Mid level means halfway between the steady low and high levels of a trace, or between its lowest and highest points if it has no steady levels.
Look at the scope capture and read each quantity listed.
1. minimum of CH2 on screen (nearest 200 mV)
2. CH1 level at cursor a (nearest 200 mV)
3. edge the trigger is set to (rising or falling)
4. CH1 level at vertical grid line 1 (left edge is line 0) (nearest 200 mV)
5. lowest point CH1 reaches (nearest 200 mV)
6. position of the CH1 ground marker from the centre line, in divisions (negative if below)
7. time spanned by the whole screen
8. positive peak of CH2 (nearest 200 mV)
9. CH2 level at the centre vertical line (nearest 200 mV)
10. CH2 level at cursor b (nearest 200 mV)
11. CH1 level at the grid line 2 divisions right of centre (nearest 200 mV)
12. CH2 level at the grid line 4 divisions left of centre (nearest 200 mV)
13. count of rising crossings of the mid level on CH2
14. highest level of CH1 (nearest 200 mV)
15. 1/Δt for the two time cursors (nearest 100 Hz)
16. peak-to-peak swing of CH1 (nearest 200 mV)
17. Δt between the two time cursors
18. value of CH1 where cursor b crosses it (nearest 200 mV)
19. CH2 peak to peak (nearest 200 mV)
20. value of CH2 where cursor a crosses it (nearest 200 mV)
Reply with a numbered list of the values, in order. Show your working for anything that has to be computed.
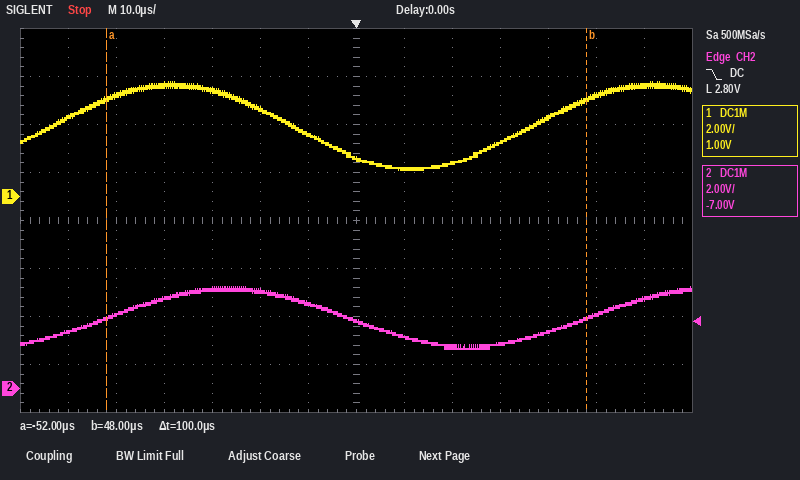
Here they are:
1. 1.6 V
2. 4.0 V
3. falling
4. 3.2 V
5. 1.2 V
6. +0.5 div
7. 140 µs
8. 4.2 V
9. 2.8 V
10. 3.0 V
11. 1.4 V
12. 3.8 V
13. 2
14. 4.8 V
15. 1 / 100 µs ≈ 10.0 kHz
16. 4.8 V − (1.2 V) = 3.6 V
17. 100 µs
18. 4.0 V
19. 4.2 V − (1.6 V) = 2.6 V
20. 3.0 V
